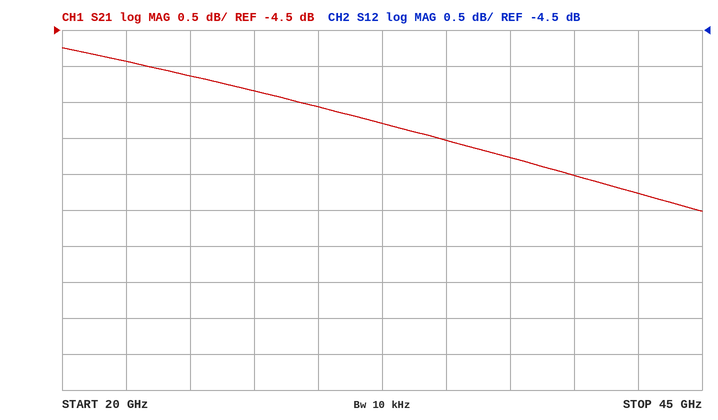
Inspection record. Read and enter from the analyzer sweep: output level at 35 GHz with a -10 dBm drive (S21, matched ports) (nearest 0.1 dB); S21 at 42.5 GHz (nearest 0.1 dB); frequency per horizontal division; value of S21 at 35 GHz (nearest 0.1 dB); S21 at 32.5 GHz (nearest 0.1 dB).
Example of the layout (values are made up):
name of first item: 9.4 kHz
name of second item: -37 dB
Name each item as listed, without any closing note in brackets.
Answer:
output level at 35 GHz with a -10 dBm drive (S21, matched ports): -16.0 dBm
S21 at 42.5 GHz: -6.8 dB
frequency per horizontal division: 2.5 GHz
value of S21 at 35 GHz: -6.0 dB
S21 at 32.5 GHz: -5.8 dB
